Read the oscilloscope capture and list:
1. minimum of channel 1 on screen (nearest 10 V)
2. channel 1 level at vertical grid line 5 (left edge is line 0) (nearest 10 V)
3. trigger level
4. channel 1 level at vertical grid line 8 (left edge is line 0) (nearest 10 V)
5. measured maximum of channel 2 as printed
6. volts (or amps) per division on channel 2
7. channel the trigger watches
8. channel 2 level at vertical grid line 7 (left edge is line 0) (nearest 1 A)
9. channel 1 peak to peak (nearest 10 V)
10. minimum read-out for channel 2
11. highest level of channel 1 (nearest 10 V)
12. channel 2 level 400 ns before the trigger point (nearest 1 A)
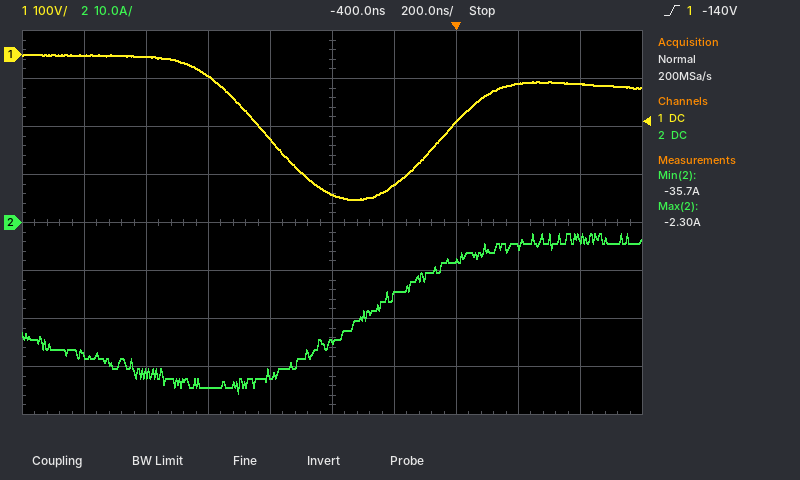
-300 V
-290 V
-140 V
-60 V
-2.30 A
10 A
channel 1
-8 A
300 V
-35.7 A
0 V
-25 A
